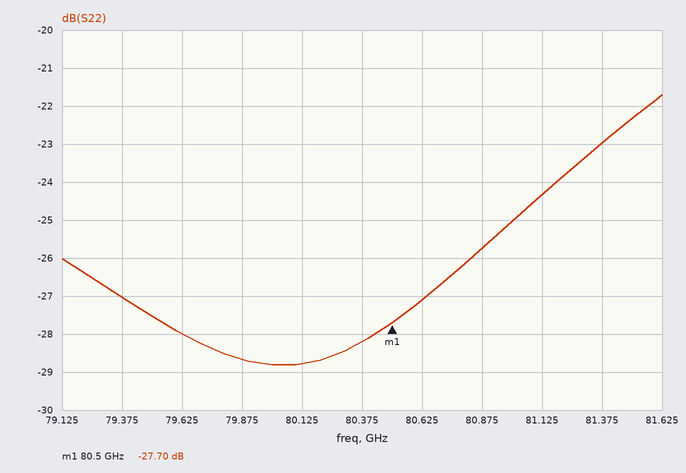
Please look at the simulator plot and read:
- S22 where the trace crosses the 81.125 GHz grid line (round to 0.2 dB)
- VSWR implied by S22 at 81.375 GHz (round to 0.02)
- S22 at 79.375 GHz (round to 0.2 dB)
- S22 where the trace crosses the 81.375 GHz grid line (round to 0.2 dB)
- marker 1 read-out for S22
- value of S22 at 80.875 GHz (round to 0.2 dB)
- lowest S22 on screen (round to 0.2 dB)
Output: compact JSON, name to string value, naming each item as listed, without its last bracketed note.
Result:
{"S22 where the trace crosses the 81.125 GHz grid line": "-24.4 dB", "VSWR implied by S22 at 81.375 GHz": "1.16", "S22 at 79.375 GHz": "-27.0 dB", "S22 where the trace crosses the 81.375 GHz grid line": "-23.0 dB", "marker 1 read-out for S22": "-27.70 dB", "value of S22 at 80.875 GHz": "-25.8 dB", "lowest S22 on screen": "-28.8 dB"}
